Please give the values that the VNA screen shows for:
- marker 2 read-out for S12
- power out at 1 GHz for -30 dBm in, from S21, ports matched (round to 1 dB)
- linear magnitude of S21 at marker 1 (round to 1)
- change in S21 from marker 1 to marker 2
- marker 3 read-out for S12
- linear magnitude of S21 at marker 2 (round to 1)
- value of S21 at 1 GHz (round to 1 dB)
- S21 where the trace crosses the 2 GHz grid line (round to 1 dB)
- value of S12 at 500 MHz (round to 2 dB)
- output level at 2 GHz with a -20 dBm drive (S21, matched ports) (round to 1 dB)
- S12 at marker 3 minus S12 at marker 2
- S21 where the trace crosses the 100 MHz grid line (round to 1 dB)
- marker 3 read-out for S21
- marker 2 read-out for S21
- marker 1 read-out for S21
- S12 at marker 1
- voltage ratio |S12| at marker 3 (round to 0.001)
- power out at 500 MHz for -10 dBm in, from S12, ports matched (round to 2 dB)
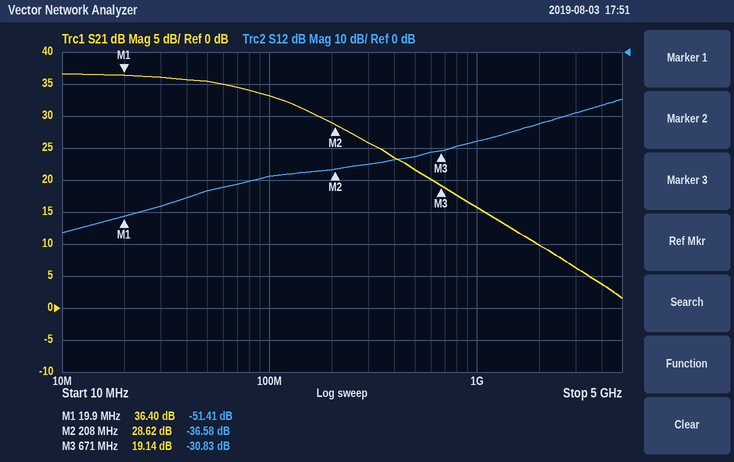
-36.58 dB
-14 dBm
66
-7.78 dB
-30.83 dB
27
16 dB
10 dB
-32 dB
-10 dBm
5.75 dB
33 dB
19.14 dB
28.62 dB
36.40 dB
-51.41 dB
0.029
-42 dBm
